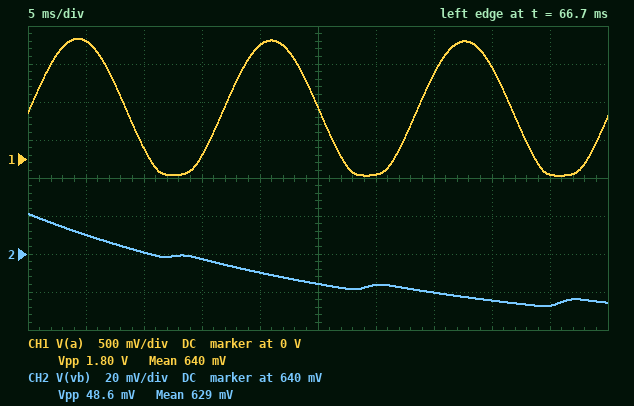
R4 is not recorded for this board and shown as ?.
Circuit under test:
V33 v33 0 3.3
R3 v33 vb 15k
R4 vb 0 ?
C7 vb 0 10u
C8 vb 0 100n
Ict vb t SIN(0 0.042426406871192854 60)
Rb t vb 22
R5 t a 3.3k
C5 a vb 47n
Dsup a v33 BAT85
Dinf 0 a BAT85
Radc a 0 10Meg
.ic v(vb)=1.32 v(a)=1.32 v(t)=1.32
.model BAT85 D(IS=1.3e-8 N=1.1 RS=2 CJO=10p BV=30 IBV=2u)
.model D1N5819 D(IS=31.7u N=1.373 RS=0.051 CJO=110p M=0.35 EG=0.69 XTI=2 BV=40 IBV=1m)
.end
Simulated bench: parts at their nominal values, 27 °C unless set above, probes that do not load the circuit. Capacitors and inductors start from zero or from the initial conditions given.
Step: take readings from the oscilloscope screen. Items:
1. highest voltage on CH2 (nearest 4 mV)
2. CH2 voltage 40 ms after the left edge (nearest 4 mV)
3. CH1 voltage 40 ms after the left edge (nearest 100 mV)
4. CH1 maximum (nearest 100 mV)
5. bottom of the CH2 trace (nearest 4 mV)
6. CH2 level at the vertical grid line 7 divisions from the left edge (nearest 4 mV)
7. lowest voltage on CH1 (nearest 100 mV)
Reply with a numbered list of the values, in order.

1. 660 mV
2. 616 mV
3. 1.2 V
4. 1.6 V
5. 612 mV
6. 620 mV
7. -200 mV
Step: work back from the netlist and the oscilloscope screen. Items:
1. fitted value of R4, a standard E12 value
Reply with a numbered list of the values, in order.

1. 3.3 kΩ
